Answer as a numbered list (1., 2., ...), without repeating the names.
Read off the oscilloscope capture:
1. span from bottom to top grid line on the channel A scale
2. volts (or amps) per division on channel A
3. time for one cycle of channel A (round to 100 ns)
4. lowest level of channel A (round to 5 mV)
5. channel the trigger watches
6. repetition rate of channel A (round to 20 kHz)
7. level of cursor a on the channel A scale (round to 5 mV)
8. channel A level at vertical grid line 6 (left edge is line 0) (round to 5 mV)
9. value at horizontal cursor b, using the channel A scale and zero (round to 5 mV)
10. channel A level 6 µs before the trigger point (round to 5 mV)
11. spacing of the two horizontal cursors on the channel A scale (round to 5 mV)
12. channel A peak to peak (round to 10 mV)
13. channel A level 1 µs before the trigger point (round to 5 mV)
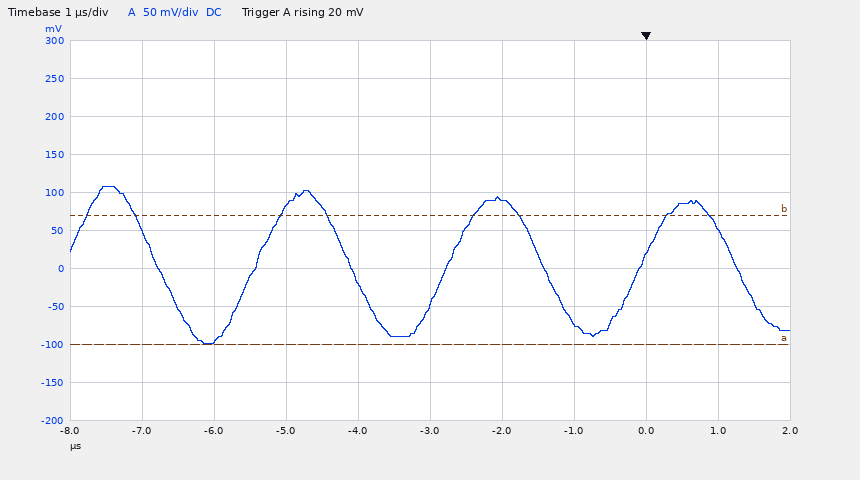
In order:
1. 500 mV
2. 50 mV
3. 2.7 µs
4. -100 mV
5. channel A
6. 380 kHz
7. -100 mV
8. 90 mV
9. 70 mV
10. -95 mV
11. 170 mV
12. 210 mV
13. -70 mV
